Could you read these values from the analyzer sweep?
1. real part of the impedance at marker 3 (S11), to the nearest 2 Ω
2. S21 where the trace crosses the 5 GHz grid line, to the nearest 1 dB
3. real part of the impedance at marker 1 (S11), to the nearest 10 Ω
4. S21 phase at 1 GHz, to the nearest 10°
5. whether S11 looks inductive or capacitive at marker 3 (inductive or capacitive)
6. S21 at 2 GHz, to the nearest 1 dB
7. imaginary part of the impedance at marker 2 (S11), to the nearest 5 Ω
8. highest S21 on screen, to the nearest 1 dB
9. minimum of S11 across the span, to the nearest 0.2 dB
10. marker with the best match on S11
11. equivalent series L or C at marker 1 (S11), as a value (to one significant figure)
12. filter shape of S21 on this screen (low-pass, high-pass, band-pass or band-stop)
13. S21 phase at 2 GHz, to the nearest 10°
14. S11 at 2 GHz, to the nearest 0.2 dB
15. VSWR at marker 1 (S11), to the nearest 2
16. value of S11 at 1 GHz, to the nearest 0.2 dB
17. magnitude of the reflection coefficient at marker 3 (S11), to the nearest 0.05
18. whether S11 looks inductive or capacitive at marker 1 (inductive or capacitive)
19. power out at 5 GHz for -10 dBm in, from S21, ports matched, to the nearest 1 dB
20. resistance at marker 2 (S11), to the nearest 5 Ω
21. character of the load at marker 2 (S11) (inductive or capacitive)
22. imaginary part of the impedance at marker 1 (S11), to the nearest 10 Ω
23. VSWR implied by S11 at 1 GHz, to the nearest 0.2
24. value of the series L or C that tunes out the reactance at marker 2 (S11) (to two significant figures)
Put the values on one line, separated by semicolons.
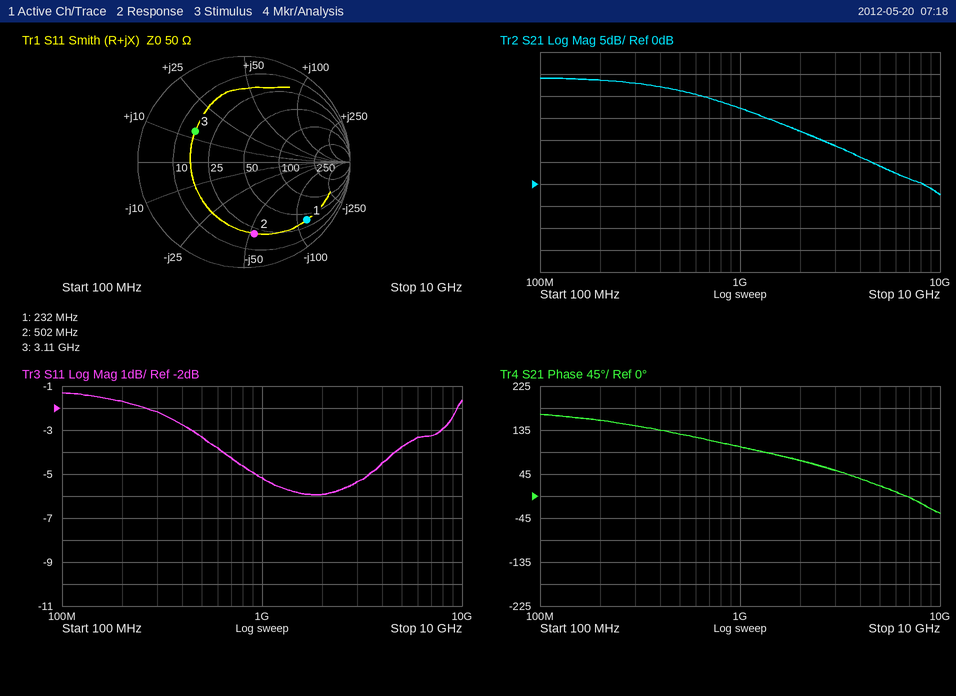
16 Ω; 4 dB; 40 Ω; 100°; inductive; 12 dB; -55 Ω; 24 dB; -6.0 dB; marker 3; 6 pF; low-pass; 70°; -6.0 dB; 10; -5.2 dB; 0.55; capacitive; -6 dBm; 20 Ω; capacitive; -120 Ω; 3.4; 17 nH
